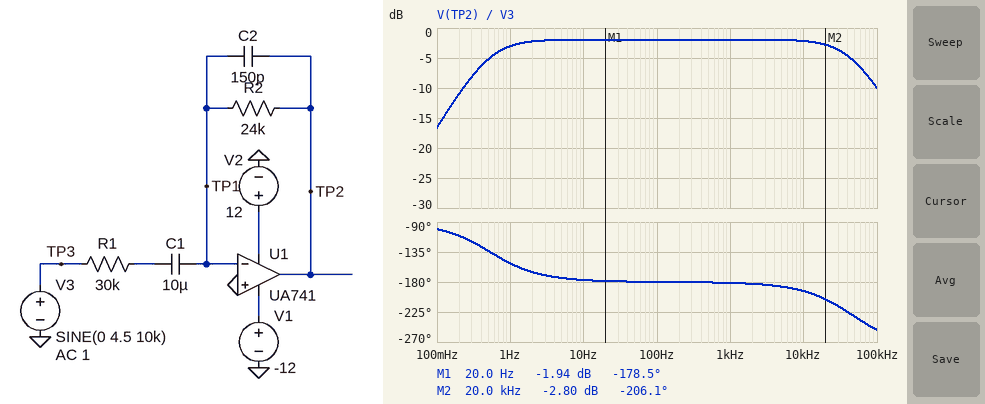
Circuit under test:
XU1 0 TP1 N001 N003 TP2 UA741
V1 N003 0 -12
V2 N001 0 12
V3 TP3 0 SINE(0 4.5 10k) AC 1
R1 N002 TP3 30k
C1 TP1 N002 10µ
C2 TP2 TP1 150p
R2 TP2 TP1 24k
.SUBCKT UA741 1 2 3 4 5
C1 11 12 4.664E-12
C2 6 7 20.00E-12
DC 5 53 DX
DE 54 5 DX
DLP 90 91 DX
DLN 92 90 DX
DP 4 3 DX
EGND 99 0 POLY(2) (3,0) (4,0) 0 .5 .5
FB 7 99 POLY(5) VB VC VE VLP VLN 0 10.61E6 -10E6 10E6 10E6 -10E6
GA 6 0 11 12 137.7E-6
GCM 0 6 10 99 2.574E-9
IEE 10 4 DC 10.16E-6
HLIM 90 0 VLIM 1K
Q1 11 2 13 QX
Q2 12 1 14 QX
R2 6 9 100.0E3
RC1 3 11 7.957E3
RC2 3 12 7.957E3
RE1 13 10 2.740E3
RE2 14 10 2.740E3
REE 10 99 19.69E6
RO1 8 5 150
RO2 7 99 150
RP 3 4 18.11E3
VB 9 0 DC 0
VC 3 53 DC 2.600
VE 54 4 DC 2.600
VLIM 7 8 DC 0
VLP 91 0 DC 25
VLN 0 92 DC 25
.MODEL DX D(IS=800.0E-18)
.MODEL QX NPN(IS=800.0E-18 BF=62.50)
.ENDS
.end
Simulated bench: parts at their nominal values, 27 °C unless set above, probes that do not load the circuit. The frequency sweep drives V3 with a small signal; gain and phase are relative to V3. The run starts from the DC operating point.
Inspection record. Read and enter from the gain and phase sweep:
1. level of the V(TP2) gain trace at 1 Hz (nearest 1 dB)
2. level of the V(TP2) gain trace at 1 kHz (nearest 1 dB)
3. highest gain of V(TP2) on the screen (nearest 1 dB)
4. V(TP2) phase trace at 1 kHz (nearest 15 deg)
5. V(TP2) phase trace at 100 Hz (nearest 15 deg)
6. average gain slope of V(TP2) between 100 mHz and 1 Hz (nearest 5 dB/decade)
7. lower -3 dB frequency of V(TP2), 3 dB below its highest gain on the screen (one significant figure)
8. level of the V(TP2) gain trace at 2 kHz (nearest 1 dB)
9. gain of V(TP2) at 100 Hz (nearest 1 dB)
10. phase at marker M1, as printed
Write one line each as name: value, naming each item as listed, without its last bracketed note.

level of the V(TP2) gain trace at 1 Hz: -3 dB
level of the V(TP2) gain trace at 1 kHz: -2 dB
highest gain of V(TP2) on the screen: -2 dB
V(TP2) phase trace at 1 kHz: -180 deg
V(TP2) phase trace at 100 Hz: -180 deg
average gain slope of V(TP2) between 100 mHz and 1 Hz: 15 dB/decade
lower -3 dB frequency of V(TP2), 3 dB below its highest gain on the screen: 500 mHz
level of the V(TP2) gain trace at 2 kHz: -2 dB
gain of V(TP2) at 100 Hz: -2 dB
phase at marker M1, as printed: -178.5 deg
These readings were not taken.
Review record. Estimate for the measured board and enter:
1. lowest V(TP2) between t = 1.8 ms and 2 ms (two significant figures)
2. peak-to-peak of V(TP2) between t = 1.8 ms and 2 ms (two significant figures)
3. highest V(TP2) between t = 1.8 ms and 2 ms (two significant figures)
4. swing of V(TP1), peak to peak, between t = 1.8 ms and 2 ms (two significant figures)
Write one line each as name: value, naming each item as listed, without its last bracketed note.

lowest V(TP2) between t = 1.8 ms and 2 ms: -3.5 V
peak-to-peak of V(TP2) between t = 1.8 ms and 2 ms: 7.0 V
highest V(TP2) between t = 1.8 ms and 2 ms: 3.5 V
swing of V(TP1), peak to peak, between t = 1.8 ms and 2 ms: 67 mV
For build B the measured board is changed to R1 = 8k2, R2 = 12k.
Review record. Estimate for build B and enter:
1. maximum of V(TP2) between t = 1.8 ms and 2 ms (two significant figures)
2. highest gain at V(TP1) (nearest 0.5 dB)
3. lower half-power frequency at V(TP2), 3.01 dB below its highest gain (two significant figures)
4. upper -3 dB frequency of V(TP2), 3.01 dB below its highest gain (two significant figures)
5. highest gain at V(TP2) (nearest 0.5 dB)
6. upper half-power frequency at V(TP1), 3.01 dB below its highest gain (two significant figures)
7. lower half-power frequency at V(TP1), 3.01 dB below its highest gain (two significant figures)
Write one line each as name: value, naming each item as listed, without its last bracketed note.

maximum of V(TP2) between t = 1.8 ms and 2 ms: 6.5 V
highest gain at V(TP1): -19.0 dB
lower half-power frequency at V(TP2), 3.01 dB below its highest gain: 1.9 Hz
upper -3 dB frequency of V(TP2), 3.01 dB below its highest gain: 79 kHz
highest gain at V(TP2): 3.5 dB
upper half-power frequency at V(TP1), 3.01 dB below its highest gain: 2.1 MHz
lower half-power frequency at V(TP1), 3.01 dB below its highest gain: 85 kHz
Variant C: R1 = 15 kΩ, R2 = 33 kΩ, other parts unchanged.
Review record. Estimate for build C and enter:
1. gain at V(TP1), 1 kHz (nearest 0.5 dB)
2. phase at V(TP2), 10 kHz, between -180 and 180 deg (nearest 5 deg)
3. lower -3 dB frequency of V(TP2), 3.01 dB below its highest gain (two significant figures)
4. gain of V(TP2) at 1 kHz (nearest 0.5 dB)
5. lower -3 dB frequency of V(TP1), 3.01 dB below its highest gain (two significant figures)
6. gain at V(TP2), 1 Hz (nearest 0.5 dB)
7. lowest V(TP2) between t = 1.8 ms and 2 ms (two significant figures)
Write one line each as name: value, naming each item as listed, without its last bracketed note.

gain at V(TP1), 1 kHz: -54.0 dB
phase at V(TP2), 10 kHz, between -180 and 180 deg: 160 deg
lower -3 dB frequency of V(TP2), 3.01 dB below its highest gain: 1.1 Hz
gain of V(TP2) at 1 kHz: 7.0 dB
lower -3 dB frequency of V(TP1), 3.01 dB below its highest gain: 33 kHz
gain at V(TP2), 1 Hz: 3.5 dB
lowest V(TP2) between t = 1.8 ms and 2 ms: -9.4 V
